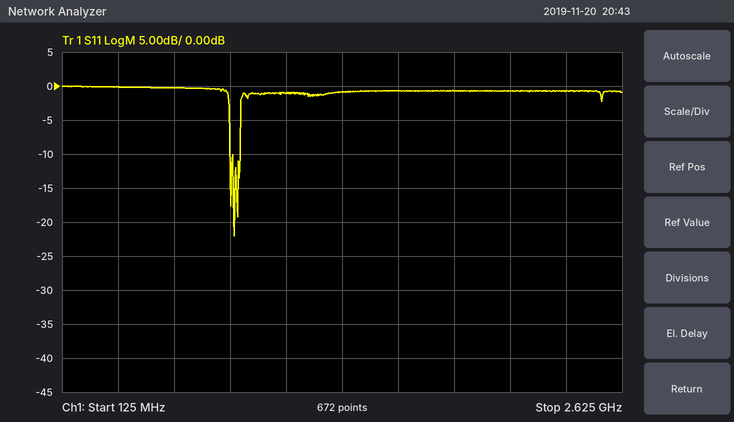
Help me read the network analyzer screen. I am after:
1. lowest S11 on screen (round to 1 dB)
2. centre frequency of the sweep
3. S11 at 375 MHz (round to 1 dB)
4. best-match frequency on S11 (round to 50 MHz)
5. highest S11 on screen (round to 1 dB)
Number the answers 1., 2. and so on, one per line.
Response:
1. -22 dB
2. 1.375 GHz
3. 0 dB
4. 900 MHz
5. 0 dB
